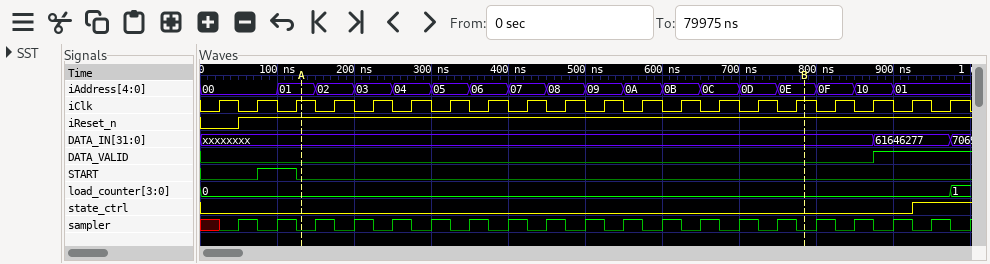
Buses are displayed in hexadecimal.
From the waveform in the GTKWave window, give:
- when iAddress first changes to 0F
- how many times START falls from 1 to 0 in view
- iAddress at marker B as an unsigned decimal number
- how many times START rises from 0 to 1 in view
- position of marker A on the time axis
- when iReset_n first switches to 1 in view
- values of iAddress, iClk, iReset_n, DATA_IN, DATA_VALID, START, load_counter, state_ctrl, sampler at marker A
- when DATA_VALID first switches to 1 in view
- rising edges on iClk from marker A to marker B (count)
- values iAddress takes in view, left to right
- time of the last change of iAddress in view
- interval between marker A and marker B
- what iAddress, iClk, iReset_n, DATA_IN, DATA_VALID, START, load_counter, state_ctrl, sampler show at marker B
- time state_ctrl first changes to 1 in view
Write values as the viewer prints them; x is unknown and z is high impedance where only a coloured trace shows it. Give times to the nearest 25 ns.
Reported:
800 ns
1
14
1
125 ns
50 ns
iAddress=01, iClk=1, iReset_n=1, DATA_IN=xxxxxxxx, DATA_VALID=0, START=0, load_counter=0, state_ctrl=0, sampler=0
875 ns
13
00, 01, 02, 03, 04, 05, 06, 07, 08, 09, 0A, 0B, 0C, 0D, 0E, 0F, 10, 01
900 ns
650 ns
iAddress=0E, iClk=1, iReset_n=1, DATA_IN=xxxxxxxx, DATA_VALID=0, START=0, load_counter=0, state_ctrl=0, sampler=0
925 ns
